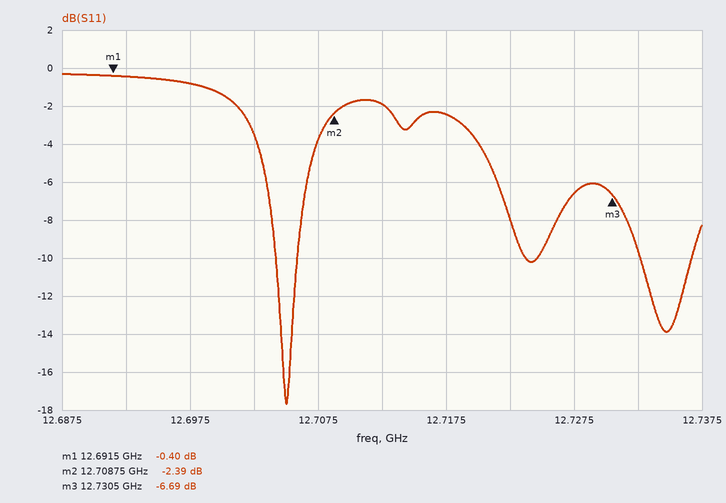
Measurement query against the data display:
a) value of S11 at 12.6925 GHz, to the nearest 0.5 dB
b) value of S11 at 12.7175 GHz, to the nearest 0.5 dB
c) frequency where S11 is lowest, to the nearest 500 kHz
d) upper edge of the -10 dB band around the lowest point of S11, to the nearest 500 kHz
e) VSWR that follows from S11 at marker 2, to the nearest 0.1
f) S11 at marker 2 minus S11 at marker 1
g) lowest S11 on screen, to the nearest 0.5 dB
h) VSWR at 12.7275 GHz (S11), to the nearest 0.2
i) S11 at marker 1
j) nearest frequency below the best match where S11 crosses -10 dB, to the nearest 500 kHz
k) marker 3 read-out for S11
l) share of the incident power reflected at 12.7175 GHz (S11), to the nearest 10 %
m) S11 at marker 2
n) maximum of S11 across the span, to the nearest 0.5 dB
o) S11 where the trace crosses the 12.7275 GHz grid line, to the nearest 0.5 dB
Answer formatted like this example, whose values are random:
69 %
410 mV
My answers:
-0.5 dB
-2.5 dB
12.7050 GHz
12.7060 GHz
7.3
-1.99 dB
-17.5 dB
2.8
-0.40 dB
12.7040 GHz
-6.69 dB
60 %
-2.39 dB
-0.5 dB
-6.5 dB
